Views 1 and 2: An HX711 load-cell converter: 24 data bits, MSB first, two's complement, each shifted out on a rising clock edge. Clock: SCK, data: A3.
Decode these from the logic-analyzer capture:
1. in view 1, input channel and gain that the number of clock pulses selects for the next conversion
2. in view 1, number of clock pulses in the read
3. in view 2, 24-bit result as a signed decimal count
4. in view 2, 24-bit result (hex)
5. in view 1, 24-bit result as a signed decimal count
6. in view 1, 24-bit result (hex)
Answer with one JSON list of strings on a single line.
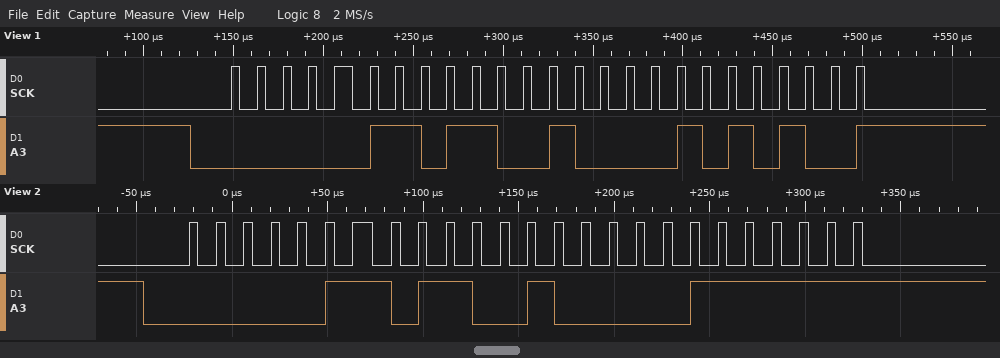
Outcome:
["channel A, gain 128", "25", "444479", "0x06C83F", "444500", "0x06C854"]
